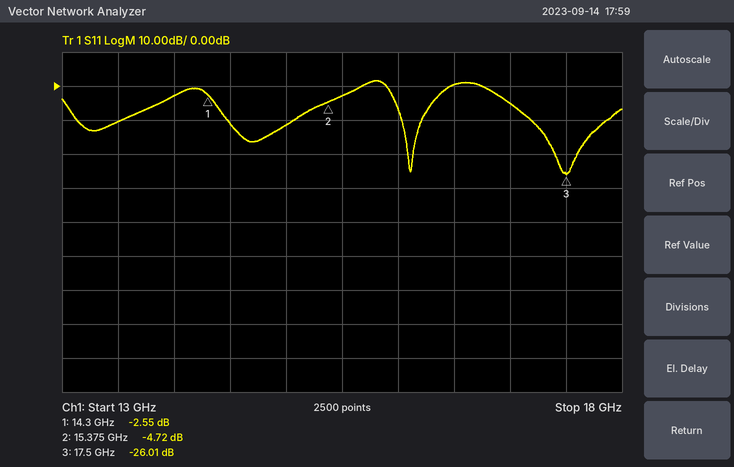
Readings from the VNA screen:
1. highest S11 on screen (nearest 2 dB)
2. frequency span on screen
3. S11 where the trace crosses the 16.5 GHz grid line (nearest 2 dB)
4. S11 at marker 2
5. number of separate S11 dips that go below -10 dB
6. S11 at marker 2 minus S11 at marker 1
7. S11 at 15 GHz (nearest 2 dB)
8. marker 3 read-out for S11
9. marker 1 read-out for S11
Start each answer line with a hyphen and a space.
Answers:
- 2 dB
- 5 GHz
- 0 dB
- -4.72 dB
- 4
- -2.17 dB
- -12 dB
- -26.01 dB
- -2.55 dB
